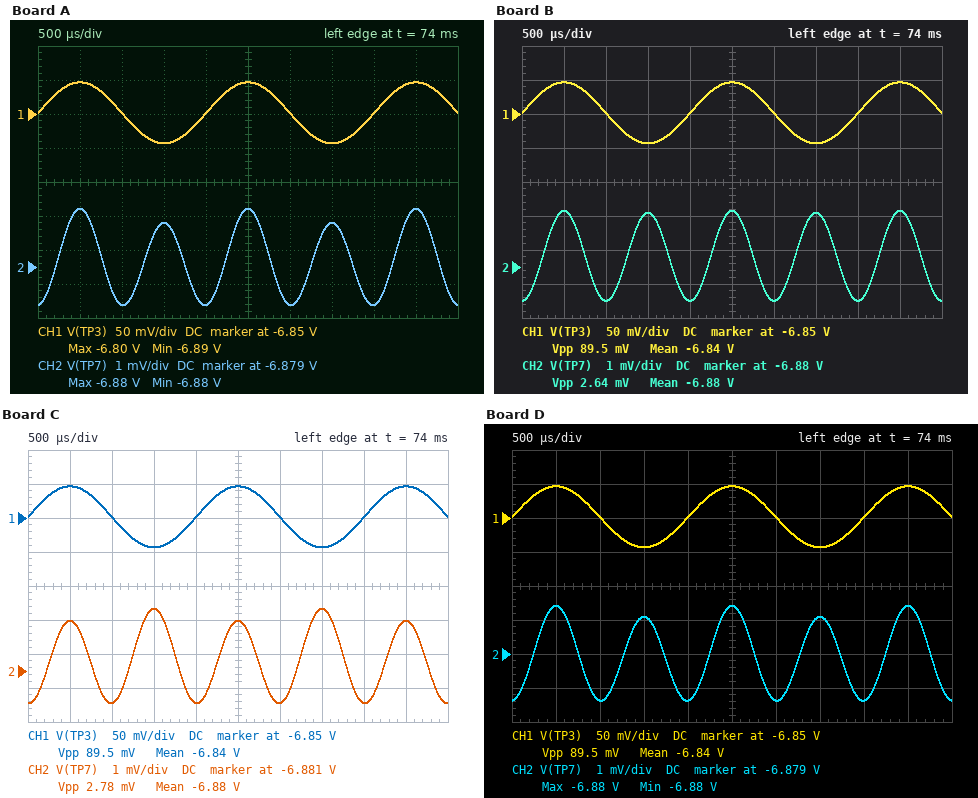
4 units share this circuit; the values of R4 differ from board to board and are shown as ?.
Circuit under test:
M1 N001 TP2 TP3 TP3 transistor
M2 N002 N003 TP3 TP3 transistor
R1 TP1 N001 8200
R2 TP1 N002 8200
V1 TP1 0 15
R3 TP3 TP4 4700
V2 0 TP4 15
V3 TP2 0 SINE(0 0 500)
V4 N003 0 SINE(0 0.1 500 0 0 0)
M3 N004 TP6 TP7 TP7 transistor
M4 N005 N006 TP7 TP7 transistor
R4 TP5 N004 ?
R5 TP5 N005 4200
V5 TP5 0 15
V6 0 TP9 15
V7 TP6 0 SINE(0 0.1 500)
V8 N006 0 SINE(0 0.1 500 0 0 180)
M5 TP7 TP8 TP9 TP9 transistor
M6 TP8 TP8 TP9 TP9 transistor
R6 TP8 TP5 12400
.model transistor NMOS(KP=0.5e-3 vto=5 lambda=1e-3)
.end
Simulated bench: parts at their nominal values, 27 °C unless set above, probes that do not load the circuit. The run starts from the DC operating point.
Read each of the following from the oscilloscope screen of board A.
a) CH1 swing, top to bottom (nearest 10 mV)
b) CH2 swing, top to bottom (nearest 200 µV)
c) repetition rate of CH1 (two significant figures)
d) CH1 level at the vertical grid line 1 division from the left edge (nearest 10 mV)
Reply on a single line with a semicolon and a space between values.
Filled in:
90 mV; 2.8 mV; 500 Hz; -6.80 V
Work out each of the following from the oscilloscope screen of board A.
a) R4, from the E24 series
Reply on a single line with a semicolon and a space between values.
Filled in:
1.8 kΩ
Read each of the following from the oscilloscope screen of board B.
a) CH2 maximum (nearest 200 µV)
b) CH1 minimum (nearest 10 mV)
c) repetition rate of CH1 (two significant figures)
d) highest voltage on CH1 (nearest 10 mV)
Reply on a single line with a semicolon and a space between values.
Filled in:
-6.8784 V; -6.89 V; 500 Hz; -6.80 V
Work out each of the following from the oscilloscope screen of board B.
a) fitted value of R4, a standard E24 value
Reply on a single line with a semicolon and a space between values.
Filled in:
3.9 kΩ
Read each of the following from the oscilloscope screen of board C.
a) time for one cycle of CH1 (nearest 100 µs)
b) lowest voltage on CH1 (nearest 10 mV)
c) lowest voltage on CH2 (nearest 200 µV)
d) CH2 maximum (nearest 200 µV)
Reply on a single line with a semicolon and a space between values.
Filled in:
2.0 ms; -6.89 V; -6.8820 V; -6.8792 V
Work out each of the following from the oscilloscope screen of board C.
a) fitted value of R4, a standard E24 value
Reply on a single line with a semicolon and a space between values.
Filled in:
6.2 kΩ
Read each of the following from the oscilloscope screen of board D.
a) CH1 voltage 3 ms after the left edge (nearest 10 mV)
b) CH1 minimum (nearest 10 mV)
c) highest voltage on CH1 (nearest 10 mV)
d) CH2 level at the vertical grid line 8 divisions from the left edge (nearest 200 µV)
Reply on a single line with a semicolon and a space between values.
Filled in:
-6.85 V; -6.89 V; -6.80 V; -6.8804 V
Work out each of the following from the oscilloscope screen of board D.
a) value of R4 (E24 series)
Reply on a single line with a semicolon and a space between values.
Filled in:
2.4 kΩ
